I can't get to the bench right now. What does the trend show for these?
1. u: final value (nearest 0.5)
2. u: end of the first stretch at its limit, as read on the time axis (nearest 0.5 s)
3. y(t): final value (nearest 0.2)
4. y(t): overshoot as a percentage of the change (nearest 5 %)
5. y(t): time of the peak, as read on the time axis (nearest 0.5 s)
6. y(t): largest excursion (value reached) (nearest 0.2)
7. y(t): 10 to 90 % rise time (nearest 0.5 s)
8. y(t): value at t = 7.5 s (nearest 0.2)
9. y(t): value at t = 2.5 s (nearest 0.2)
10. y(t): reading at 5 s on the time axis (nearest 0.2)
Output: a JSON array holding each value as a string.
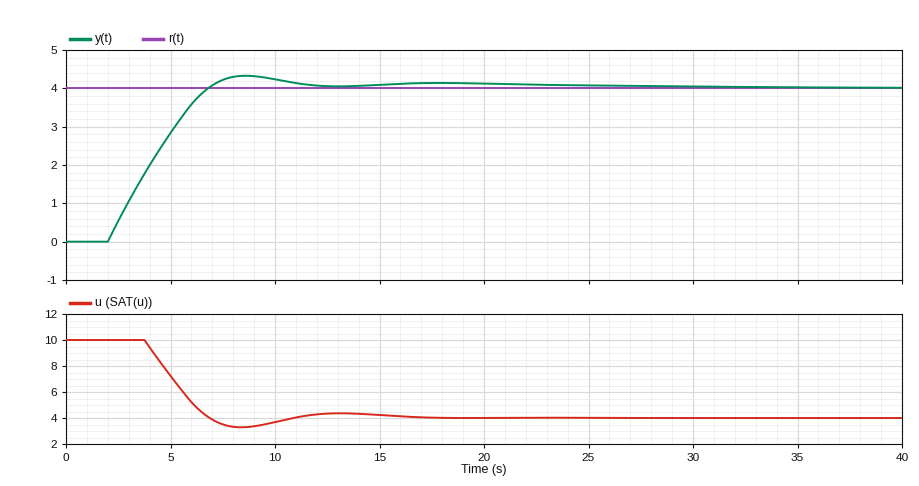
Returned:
["4.0", "4.0 s", "4.0", "10 %", "8.5 s", "4.4", "3.5 s", "4.2", "0.6", "2.8"]
